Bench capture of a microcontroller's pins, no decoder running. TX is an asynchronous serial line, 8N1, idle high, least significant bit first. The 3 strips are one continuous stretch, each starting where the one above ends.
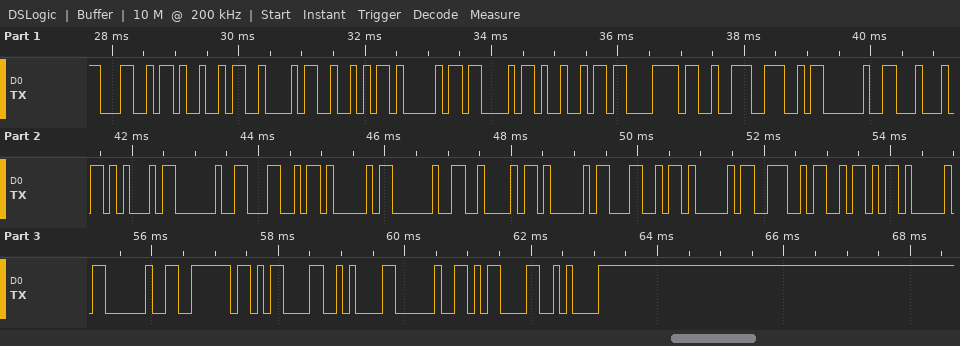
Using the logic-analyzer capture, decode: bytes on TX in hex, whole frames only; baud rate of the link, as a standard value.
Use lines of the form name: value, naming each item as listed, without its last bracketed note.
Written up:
bytes on TX in hex, whole frames only: 4C 49 42 52 41 43 49 C3 93 4E 20 44 45 20 4C 41 20 42 41 4C 41 4E 5A 41 20 7E 0D 0A 20 0D 0A
baud rate of the link, as a standard value: 9600 baud
